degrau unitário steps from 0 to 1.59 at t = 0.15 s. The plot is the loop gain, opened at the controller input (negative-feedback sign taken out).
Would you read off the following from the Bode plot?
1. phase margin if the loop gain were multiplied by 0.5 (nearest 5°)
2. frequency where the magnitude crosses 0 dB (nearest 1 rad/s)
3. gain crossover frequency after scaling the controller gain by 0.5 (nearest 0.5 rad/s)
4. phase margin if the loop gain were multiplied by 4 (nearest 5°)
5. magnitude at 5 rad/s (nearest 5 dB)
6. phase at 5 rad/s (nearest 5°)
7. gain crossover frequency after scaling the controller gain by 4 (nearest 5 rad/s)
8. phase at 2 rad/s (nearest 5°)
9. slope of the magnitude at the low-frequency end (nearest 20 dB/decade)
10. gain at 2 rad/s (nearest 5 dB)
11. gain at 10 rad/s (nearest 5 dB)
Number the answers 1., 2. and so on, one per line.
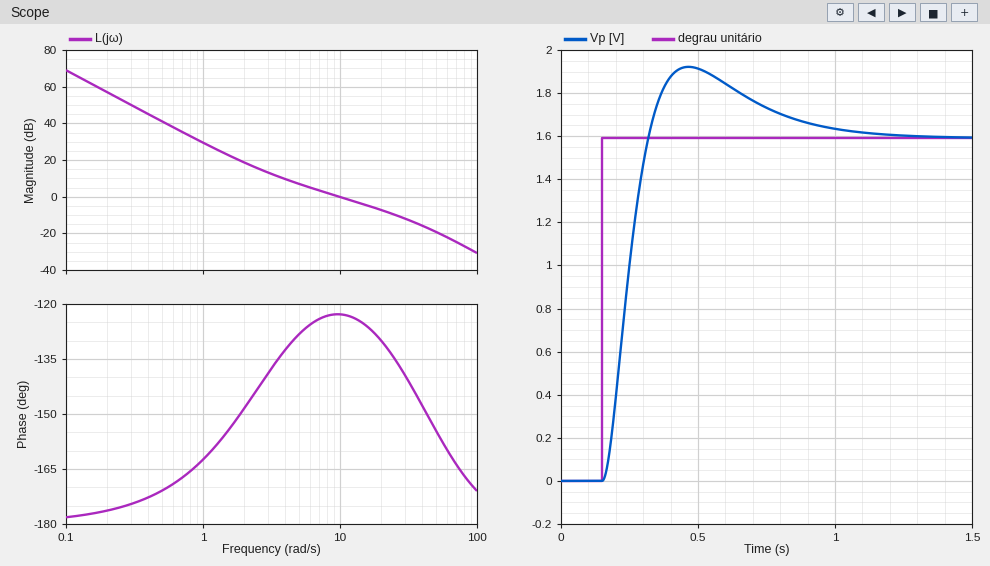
1. 55°
2. 10 rad/s
3. 5.5 rad/s
4. 40°
5. 5 dB
6. -130°
7. 30 rad/s
8. -150°
9. -40 dB/decade
10. 20 dB
11. 0 dB
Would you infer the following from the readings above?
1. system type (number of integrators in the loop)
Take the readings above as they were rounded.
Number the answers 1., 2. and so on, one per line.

1. 2
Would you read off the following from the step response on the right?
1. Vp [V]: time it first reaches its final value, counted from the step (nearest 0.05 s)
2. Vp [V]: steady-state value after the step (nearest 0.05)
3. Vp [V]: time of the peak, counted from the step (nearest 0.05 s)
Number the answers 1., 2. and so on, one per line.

1. 0.15 s
2. 1.60
3. 0.30 s
